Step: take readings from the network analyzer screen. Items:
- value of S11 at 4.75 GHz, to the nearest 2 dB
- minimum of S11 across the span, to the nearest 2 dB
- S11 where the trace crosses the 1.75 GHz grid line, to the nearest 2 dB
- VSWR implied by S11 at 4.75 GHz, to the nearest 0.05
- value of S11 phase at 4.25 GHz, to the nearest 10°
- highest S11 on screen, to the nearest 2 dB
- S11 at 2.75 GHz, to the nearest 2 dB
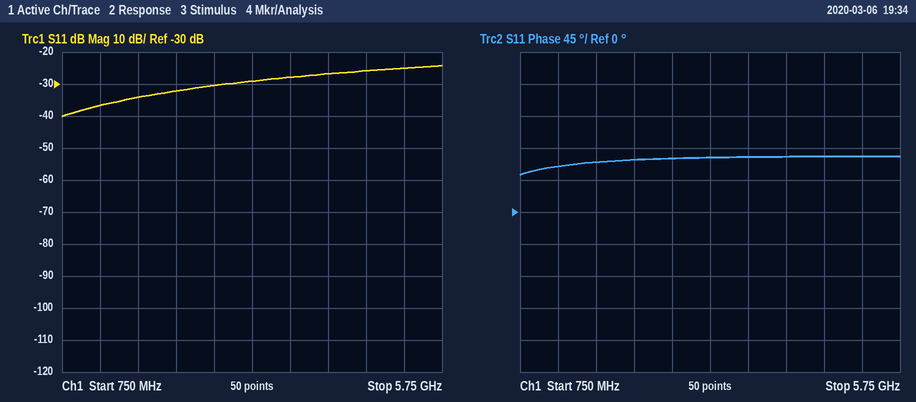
-26 dB
-40 dB
-34 dB
1.10
80°
-24 dB
-30 dB
